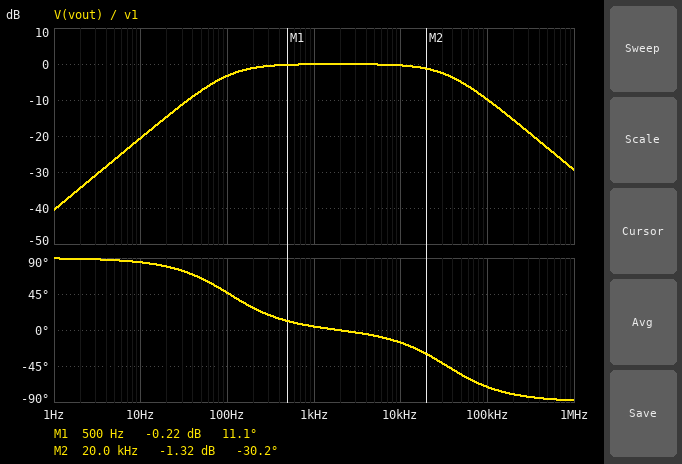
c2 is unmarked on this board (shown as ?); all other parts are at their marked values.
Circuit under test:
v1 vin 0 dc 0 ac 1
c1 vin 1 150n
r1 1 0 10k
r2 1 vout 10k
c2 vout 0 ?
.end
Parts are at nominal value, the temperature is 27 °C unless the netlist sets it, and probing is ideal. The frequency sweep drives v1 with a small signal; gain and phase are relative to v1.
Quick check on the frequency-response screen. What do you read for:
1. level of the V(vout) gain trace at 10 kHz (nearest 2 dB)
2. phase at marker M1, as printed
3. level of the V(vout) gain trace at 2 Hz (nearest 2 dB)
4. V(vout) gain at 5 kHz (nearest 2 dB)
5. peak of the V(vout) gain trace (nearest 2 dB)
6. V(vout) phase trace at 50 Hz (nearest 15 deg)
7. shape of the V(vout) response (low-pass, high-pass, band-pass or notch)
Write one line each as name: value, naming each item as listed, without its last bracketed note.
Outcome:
level of the V(vout) gain trace at 10 kHz: 0 dB
phase at marker M1, as printed: 11.1 deg
level of the V(vout) gain trace at 2 Hz: -34 dB
V(vout) gain at 5 kHz: 0 dB
peak of the V(vout) gain trace: 0 dB
V(vout) phase trace at 50 Hz: 60 deg
shape of the V(vout) response: band-pass
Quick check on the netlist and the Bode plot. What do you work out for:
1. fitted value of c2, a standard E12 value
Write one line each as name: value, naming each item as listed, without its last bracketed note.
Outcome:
fitted value of c2, a standard E12 value: 470 pF
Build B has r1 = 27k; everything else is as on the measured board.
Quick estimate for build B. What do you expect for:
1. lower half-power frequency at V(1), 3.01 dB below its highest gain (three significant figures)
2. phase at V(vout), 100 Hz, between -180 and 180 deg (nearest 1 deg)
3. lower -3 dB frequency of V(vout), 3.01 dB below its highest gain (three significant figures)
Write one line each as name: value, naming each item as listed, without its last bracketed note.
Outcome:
lower half-power frequency at V(1), 3.01 dB below its highest gain: 39.4 Hz
phase at V(vout), 100 Hz, between -180 and 180 deg: 21 deg
lower -3 dB frequency of V(vout), 3.01 dB below its highest gain: 39.1 Hz
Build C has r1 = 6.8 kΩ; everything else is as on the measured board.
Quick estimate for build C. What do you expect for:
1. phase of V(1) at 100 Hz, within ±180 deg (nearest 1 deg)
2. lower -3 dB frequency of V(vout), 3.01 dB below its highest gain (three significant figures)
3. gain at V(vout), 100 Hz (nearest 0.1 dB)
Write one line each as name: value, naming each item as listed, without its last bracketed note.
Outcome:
phase of V(1) at 100 Hz, within ±180 deg: 57 deg
lower -3 dB frequency of V(vout), 3.01 dB below its highest gain: 154 Hz
gain at V(vout), 100 Hz: -5.4 dB
